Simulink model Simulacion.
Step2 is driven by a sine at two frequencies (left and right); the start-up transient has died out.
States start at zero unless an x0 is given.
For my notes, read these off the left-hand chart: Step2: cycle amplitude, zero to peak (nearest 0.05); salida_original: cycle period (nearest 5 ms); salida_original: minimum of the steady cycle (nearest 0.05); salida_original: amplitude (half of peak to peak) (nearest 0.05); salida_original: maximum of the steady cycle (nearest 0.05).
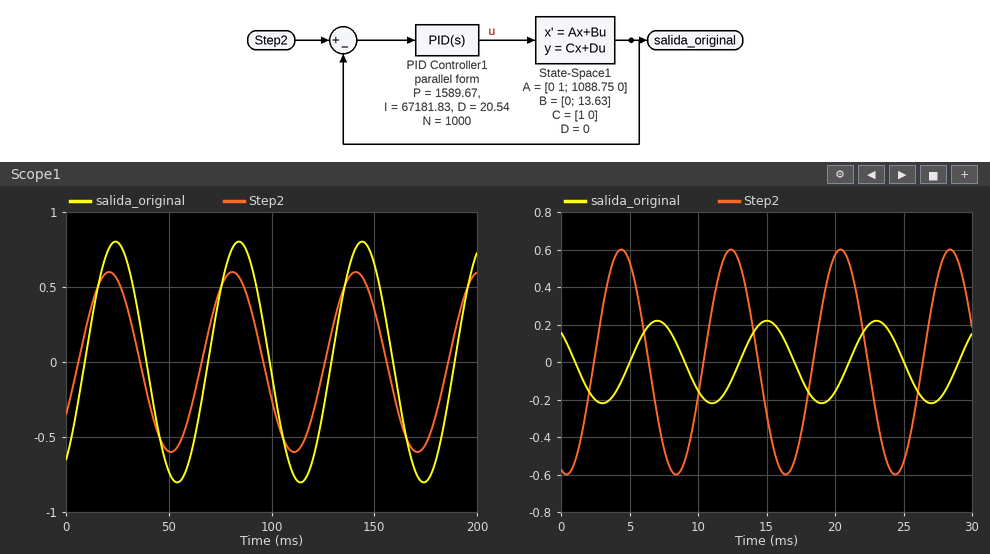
0.60
60 ms
-0.80
0.80
0.80
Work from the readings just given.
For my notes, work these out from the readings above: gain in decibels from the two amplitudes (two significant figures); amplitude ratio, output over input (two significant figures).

2.5 dB
1.3
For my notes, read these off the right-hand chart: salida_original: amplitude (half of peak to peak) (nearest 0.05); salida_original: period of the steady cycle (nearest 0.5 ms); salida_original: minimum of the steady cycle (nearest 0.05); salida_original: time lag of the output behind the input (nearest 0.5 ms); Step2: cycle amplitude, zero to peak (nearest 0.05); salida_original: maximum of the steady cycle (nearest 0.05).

0.20
8.0 ms
-0.20
2.5 ms
0.60
0.20
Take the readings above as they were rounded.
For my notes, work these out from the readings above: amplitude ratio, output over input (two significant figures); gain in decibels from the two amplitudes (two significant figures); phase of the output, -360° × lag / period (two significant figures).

0.33
-9.5 dB
-110°
